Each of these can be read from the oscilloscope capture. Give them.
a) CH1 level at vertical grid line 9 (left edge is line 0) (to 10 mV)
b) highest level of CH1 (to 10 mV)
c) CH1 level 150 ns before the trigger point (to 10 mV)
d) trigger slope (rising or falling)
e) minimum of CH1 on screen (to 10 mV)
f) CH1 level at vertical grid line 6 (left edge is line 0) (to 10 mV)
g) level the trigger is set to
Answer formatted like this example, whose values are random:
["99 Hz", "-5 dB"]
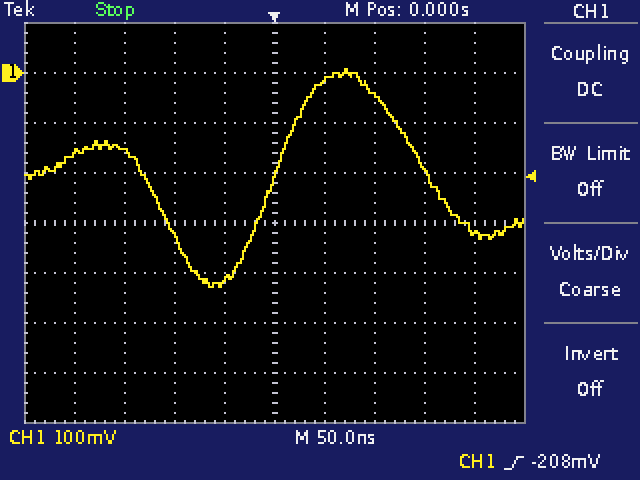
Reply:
["-320 mV", "10 mV", "-160 mV", "rising", "-430 mV", "-20 mV", "-208 mV"]
